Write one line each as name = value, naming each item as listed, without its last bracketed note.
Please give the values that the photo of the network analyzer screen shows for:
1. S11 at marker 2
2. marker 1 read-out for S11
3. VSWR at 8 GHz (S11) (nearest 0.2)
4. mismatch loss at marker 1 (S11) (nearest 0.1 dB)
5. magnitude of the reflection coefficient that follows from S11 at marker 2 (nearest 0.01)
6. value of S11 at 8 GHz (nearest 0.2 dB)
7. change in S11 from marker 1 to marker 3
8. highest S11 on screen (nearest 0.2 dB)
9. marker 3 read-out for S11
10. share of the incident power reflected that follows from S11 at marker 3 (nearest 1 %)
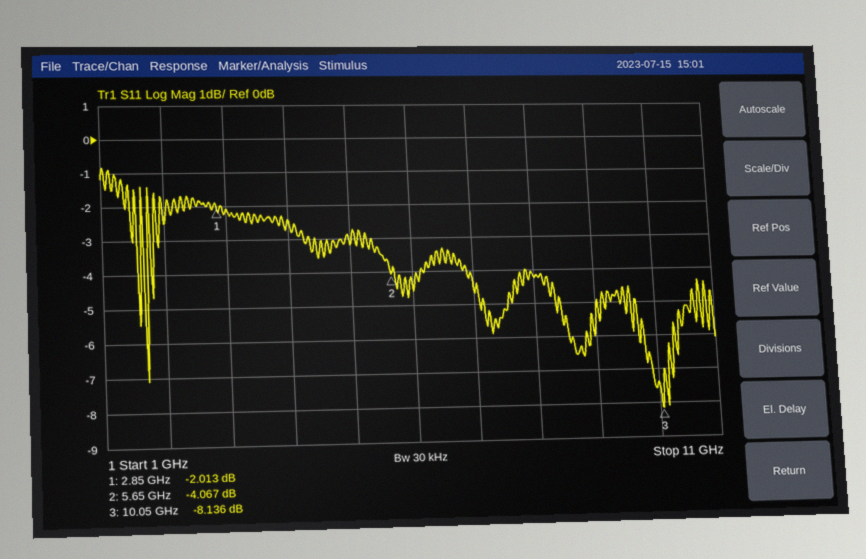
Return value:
S11 at marker 2 = -4.067 dB
marker 1 read-out for S11 = -2.013 dB
VSWR at 8 GHz (S11) = 4.2
mismatch loss at marker 1 (S11) = 4.3 dB
magnitude of the reflection coefficient that follows from S11 at marker 2 = 0.63
value of S11 at 8 GHz = -4.2 dB
change in S11 from marker 1 to marker 3 = -6.123 dB
highest S11 on screen = -0.8 dB
marker 3 read-out for S11 = -8.136 dB
share of the incident power reflected that follows from S11 at marker 3 = 15 %
